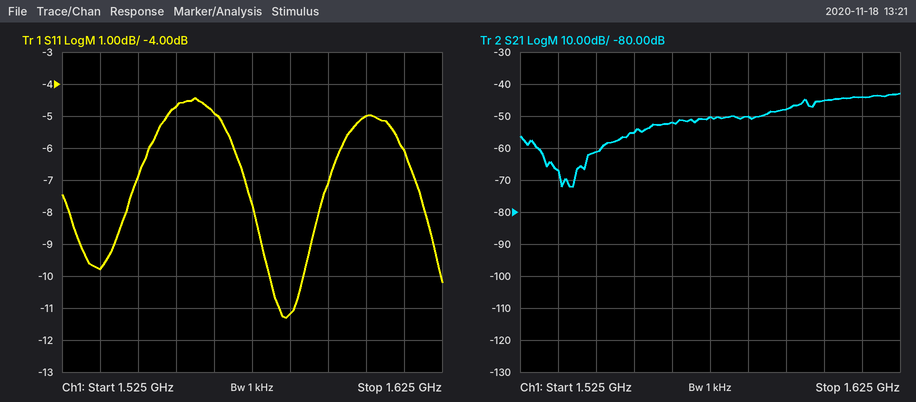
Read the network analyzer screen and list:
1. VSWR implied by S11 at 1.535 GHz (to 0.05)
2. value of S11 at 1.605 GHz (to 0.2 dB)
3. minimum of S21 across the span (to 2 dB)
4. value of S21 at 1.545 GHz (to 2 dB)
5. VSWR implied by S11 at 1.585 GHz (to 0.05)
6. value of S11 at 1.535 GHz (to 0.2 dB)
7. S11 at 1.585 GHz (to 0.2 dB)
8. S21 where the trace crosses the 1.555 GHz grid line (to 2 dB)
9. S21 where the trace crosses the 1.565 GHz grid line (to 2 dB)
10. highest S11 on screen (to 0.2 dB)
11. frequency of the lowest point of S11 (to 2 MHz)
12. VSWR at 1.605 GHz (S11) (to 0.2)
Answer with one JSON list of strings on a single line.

["1.95", "-5.0 dB", "-72 dB", "-62 dB", "1.75", "-9.8 dB", "-11.2 dB", "-56 dB", "-52 dB", "-4.4 dB", "1.584 GHz", "3.6"]
